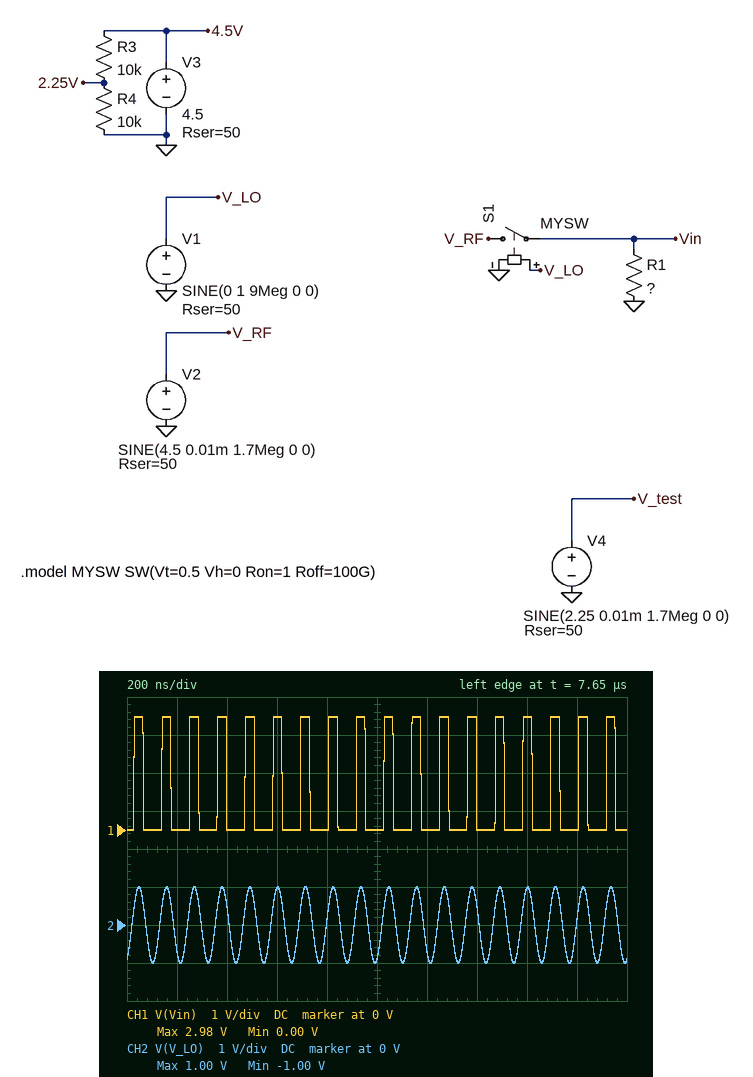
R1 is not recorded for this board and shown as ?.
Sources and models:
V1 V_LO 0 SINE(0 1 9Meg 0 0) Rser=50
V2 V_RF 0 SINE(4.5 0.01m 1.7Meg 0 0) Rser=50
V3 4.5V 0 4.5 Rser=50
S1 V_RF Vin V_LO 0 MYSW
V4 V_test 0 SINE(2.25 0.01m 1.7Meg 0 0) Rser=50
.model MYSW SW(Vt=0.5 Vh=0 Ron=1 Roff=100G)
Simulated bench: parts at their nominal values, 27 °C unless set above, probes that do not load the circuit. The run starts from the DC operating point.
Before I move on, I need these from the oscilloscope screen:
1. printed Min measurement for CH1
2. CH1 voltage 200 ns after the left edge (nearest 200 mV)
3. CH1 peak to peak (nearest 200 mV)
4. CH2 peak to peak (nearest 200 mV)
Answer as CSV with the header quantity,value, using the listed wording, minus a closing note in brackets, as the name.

quantity,value
printed Min measurement for CH1,0.00 V
CH1 voltage 200 ns after the left edge,0 V
CH1 peak to peak,3.0 V
CH2 peak to peak,2.0 V
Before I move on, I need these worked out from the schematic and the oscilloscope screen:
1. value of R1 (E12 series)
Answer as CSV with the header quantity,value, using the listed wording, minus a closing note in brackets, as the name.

quantity,value
value of R1,100 Ω
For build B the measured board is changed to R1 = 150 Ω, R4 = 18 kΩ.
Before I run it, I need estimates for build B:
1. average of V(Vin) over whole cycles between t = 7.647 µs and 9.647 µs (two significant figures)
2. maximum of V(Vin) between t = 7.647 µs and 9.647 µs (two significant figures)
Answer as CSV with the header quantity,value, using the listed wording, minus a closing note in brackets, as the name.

quantity,value
average of V(Vin) over whole cycles between t = 7.647 µs and 9.647 µs,1.1 V
maximum of V(Vin) between t = 7.647 µs and 9.647 µs,3.4 V
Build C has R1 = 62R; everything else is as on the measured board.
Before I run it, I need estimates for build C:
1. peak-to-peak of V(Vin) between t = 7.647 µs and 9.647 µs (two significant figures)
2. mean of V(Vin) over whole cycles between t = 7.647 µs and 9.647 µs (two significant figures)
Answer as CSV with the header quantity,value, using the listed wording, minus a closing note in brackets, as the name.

quantity,value
peak-to-peak of V(Vin) between t = 7.647 µs and 9.647 µs,2.5 V
mean of V(Vin) over whole cycles between t = 7.647 µs and 9.647 µs,820 mV
